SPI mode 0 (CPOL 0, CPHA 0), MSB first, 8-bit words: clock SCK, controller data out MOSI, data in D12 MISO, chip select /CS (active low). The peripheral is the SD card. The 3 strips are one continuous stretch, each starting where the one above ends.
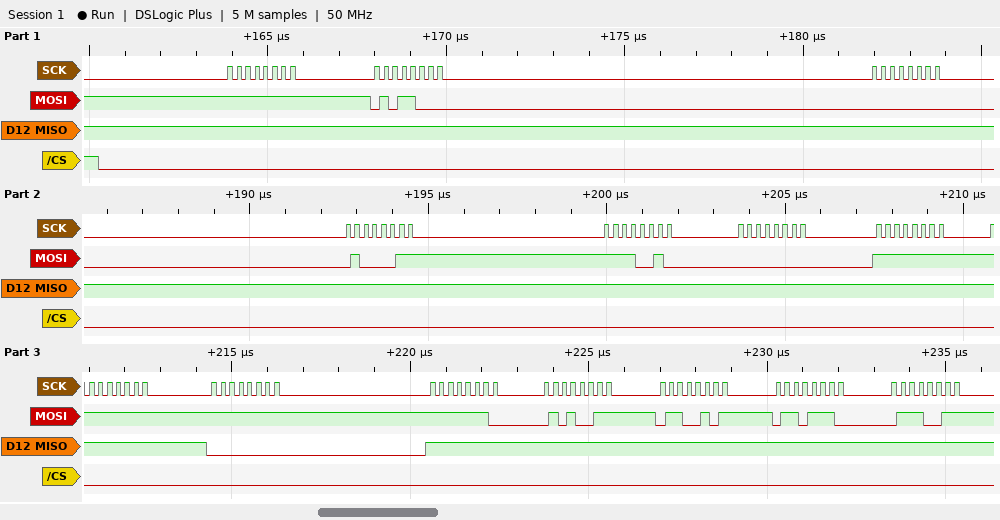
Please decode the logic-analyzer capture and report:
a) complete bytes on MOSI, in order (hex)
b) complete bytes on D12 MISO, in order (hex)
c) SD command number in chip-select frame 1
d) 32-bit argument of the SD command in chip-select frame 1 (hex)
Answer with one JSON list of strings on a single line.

["FF 58 00 43 F2 00 FF FF FF FE 53 65 6E 73", "FF FF FF FF FF FF FF FF 00 FF FF FF FF FF", "CMD24", "0x0043F200"]
